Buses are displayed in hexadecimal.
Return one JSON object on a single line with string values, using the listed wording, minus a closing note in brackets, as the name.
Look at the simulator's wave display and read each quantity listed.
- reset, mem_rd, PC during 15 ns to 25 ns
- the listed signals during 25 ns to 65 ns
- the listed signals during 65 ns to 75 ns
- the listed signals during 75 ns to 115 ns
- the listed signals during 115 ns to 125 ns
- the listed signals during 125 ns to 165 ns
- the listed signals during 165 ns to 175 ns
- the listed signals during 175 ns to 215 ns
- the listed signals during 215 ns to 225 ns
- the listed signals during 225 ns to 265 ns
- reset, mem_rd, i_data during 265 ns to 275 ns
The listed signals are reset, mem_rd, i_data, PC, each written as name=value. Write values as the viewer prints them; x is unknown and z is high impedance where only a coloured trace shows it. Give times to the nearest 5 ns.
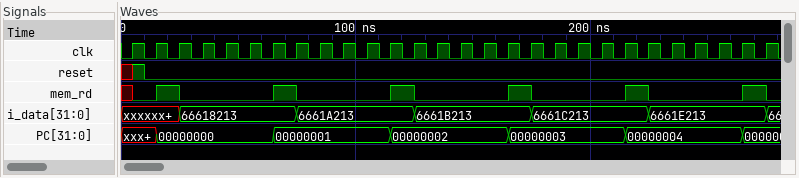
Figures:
{"reset, mem_rd, PC during 15 ns to 25 ns": "reset=0, mem_rd=1, PC=00000000", "the listed signals during 25 ns to 65 ns": "reset=0, mem_rd=0, i_data=66618213, PC=00000000", "the listed signals during 65 ns to 75 ns": "reset=0, mem_rd=1, i_data=66618213, PC=00000001", "the listed signals during 75 ns to 115 ns": "reset=0, mem_rd=0, i_data=6661A213, PC=00000001", "the listed signals during 115 ns to 125 ns": "reset=0, mem_rd=1, i_data=6661A213, PC=00000002", "the listed signals during 125 ns to 165 ns": "reset=0, mem_rd=0, i_data=6661B213, PC=00000002", "the listed signals during 165 ns to 175 ns": "reset=0, mem_rd=1, i_data=6661B213, PC=00000003", "the listed signals during 175 ns to 215 ns": "reset=0, mem_rd=0, i_data=6661C213, PC=00000003", "the listed signals during 215 ns to 225 ns": "reset=0, mem_rd=1, i_data=6661C213, PC=00000004", "the listed signals during 225 ns to 265 ns": "reset=0, mem_rd=0, i_data=6661E213, PC=00000004", "reset, mem_rd, i_data during 265 ns to 275 ns": "reset=0, mem_rd=1, i_data=6661E213"}
